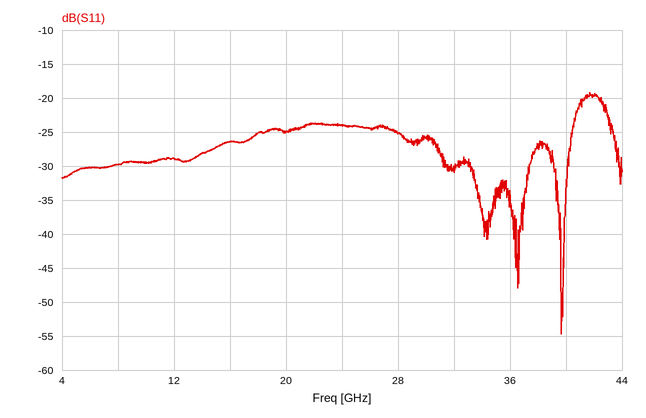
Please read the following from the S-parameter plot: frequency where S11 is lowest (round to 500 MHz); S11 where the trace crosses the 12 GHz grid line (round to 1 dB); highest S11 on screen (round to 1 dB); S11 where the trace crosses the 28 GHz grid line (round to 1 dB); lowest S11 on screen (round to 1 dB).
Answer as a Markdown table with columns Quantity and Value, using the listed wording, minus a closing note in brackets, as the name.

| Quantity | Value |
|---|---|
| frequency where S11 is lowest | 39.5 GHz |
| S11 where the trace crosses the 12 GHz grid line | -29 dB |
| highest S11 on screen | -19 dB |
| S11 where the trace crosses the 28 GHz grid line | -25 dB |
| lowest S11 on screen | -55 dB |
